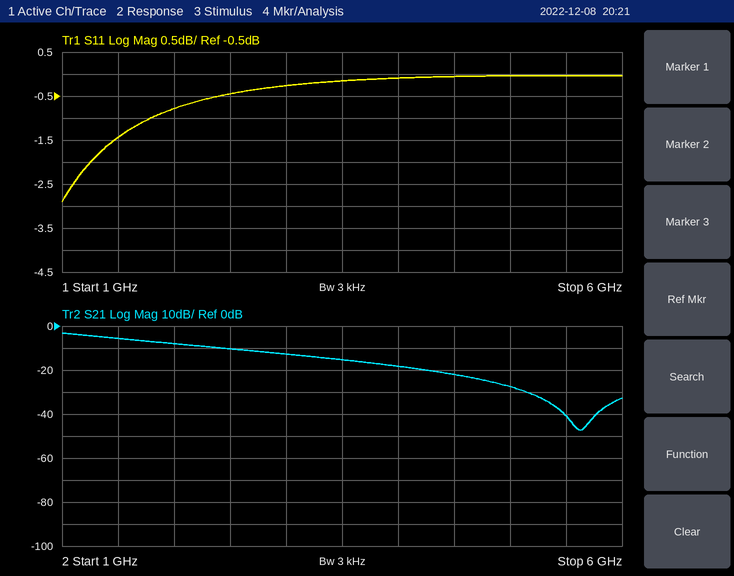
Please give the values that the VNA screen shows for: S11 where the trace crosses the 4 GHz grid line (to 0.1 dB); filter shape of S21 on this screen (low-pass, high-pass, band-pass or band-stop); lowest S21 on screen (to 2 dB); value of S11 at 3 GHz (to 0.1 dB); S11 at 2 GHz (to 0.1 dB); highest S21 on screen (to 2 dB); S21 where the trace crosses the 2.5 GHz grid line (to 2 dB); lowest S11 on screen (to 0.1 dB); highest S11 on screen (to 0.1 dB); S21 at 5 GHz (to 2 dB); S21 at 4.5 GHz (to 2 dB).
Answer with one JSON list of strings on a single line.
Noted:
["-0.1 dB", "low-pass", "-48 dB", "-0.3 dB", "-0.8 dB", "-4 dB", "-10 dB", "-2.9 dB", "0.0 dB", "-28 dB", "-22 dB"]
